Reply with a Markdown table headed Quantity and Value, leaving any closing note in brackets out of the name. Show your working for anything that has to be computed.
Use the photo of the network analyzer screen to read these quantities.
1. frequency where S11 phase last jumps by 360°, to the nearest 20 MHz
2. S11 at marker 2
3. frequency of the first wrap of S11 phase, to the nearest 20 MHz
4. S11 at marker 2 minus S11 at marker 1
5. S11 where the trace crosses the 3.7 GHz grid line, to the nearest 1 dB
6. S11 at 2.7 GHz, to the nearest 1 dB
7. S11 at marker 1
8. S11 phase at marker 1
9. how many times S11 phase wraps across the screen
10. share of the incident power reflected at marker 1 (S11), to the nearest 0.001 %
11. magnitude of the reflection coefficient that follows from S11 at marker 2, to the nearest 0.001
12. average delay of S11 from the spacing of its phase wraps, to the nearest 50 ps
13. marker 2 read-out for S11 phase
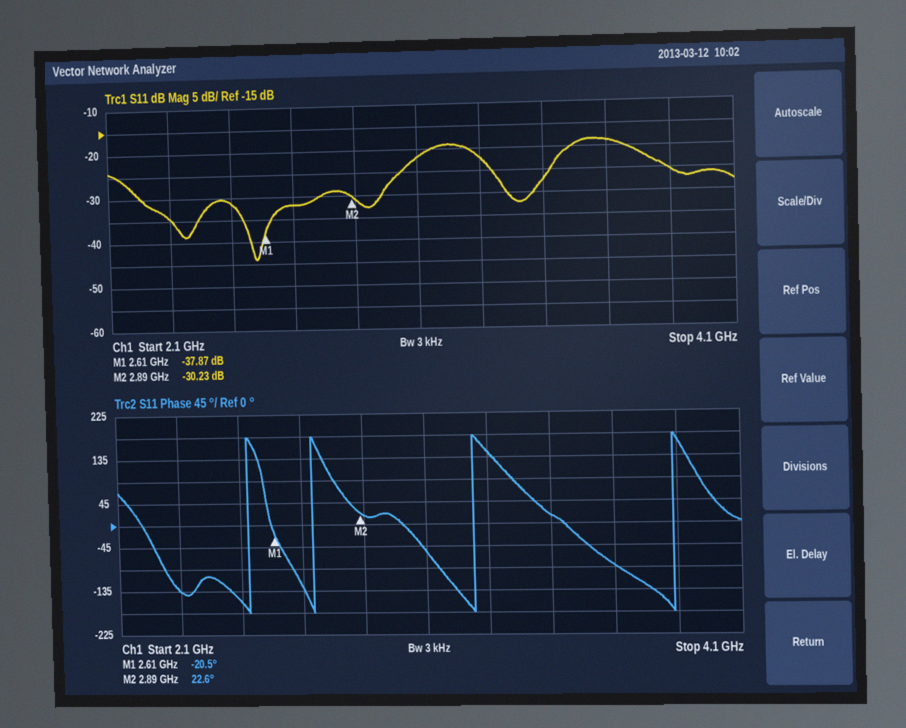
| Quantity | Value |
|---|---|
| frequency where S11 phase last jumps by 360°, to the nearest 20 MHz | 3.88 GHz |
| S11 at marker 2 | -30.23 dB |
| frequency of the first wrap of S11 phase, to the nearest 20 MHz | 2.52 GHz |
| S11 at marker 2 minus S11 at marker 1 | -30.23 − (-37.87) = 7.64 dB |
| S11 where the trace crosses the 3.7 GHz grid line, to the nearest 1 dB | -19 dB |
| S11 at 2.7 GHz, to the nearest 1 dB | -32 dB |
| S11 at marker 1 | -37.87 dB |
| S11 phase at marker 1 | -20.5° |
| how many times S11 phase wraps across the screen | 4 |
| share of the incident power reflected at marker 1 (S11), to the nearest 0.001 % | 10^(-37.87/10) ≈ 0.016 % |
| magnitude of the reflection coefficient that follows from S11 at marker 2, to the nearest 0.001 | 10^(-30.23/20) ≈ 0.031 |
| average delay of S11 from the spacing of its phase wraps, to the nearest 50 ps | 3 cycles / (3.88 GHz − 2.52 GHz) ≈ 2.21 ns, so 2.20 ns to the nearest 50 ps |
| marker 2 read-out for S11 phase | 22.6° |
